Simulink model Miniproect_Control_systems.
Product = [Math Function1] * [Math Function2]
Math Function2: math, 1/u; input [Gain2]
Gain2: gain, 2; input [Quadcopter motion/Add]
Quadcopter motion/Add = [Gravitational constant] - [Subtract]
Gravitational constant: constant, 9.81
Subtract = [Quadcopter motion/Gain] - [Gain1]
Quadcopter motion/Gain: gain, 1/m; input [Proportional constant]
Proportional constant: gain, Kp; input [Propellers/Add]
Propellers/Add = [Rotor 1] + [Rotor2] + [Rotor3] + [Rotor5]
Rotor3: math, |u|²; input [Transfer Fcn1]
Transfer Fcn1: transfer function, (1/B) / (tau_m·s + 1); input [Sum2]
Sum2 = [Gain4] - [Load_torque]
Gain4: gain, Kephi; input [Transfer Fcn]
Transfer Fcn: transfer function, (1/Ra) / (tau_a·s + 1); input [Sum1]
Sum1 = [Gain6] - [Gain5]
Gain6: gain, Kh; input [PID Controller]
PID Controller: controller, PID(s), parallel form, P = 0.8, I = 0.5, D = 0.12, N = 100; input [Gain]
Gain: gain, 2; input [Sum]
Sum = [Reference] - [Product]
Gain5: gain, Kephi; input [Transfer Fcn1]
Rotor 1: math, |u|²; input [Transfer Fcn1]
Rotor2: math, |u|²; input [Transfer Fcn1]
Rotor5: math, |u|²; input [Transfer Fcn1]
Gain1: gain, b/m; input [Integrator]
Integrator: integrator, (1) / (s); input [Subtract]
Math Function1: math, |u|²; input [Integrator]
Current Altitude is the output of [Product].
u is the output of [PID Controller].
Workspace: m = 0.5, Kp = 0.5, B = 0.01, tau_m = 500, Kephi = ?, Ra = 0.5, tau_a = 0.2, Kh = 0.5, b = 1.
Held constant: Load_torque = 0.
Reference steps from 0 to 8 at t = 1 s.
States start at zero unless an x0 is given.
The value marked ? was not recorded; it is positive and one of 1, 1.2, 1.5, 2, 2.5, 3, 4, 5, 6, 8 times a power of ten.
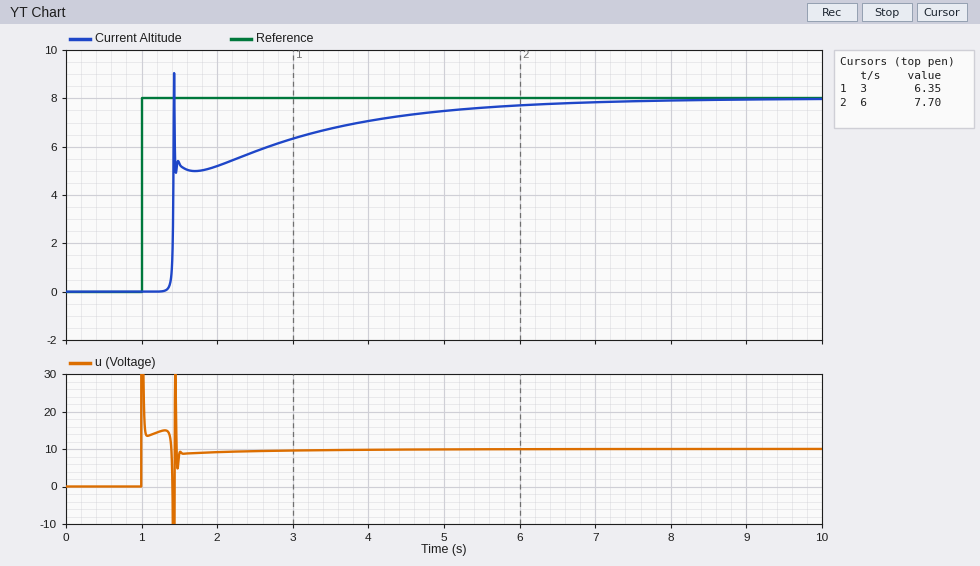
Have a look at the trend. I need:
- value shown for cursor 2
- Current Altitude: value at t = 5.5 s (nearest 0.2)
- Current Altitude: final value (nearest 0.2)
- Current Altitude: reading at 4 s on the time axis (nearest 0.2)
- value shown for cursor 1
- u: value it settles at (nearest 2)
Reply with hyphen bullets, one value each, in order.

- 7.70
- 7.6
- 8.0
- 7.0
- 6.35
- 10
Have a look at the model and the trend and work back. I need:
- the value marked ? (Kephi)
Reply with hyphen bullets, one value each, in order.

- 2
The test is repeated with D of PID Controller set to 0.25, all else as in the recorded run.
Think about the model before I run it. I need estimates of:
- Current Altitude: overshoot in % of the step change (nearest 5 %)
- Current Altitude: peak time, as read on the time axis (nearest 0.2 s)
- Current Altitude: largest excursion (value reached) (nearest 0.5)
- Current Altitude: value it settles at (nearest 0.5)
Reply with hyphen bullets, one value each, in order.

- 10 %
- 1.2 s
- 9.0
- 8.0
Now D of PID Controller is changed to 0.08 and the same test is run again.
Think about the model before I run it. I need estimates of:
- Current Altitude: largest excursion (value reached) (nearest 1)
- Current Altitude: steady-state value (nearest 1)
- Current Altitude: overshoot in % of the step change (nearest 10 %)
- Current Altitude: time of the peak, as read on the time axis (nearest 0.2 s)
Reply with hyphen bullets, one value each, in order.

- 14
- 8
- 80 %
- 1.4 s
